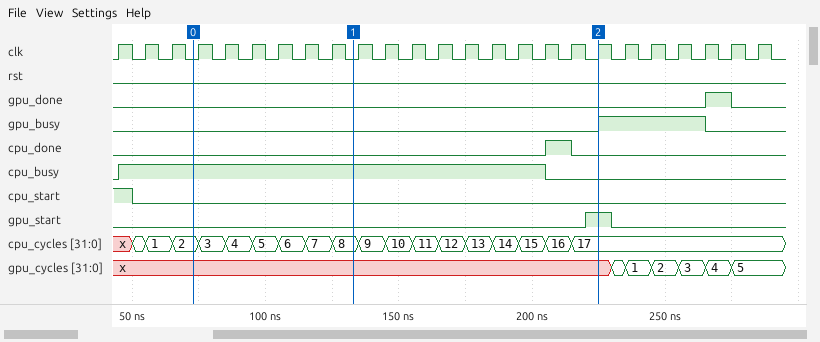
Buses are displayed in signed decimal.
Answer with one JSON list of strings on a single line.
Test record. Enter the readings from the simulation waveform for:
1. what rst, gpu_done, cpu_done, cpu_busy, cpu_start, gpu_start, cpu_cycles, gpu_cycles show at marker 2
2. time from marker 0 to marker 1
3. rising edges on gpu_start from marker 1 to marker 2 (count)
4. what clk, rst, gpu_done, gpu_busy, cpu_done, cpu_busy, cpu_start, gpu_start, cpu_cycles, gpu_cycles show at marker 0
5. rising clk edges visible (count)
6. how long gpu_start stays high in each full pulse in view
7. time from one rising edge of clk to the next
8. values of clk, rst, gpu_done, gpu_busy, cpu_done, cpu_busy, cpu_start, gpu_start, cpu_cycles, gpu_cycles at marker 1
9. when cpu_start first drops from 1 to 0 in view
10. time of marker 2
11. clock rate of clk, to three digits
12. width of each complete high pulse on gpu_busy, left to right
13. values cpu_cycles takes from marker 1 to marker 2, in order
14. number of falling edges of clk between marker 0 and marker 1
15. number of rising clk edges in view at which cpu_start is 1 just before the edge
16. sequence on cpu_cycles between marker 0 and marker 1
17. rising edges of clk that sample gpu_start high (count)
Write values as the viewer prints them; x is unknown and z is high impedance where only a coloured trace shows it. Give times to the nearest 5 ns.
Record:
["rst=0, gpu_done=0, cpu_done=0, cpu_busy=0, cpu_start=0, gpu_start=1, cpu_cycles=17, gpu_cycles=x", "60 ns", "1", "clk=0, rst=0, gpu_done=0, gpu_busy=0, cpu_done=0, cpu_busy=1, cpu_start=0, gpu_start=0, cpu_cycles=2, gpu_cycles=x", "25", "10 ns", "10 ns", "clk=0, rst=0, gpu_done=0, gpu_busy=0, cpu_done=0, cpu_busy=1, cpu_start=0, gpu_start=0, cpu_cycles=8, gpu_cycles=x", "50 ns", "225 ns", "100 MHz", "40 ns", "8, 9, 10, 11, 12, 13, 14, 15, 16, 17", "6", "1", "2, 3, 4, 5, 6, 7, 8", "1"]
